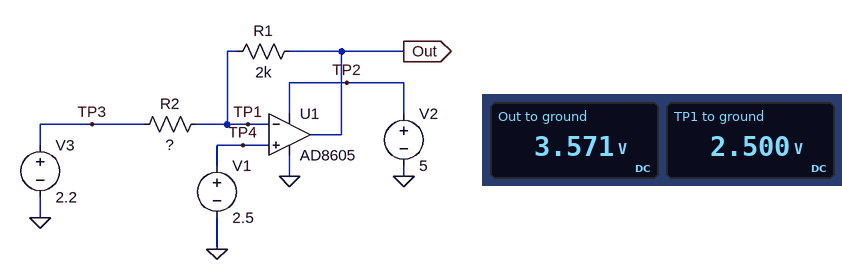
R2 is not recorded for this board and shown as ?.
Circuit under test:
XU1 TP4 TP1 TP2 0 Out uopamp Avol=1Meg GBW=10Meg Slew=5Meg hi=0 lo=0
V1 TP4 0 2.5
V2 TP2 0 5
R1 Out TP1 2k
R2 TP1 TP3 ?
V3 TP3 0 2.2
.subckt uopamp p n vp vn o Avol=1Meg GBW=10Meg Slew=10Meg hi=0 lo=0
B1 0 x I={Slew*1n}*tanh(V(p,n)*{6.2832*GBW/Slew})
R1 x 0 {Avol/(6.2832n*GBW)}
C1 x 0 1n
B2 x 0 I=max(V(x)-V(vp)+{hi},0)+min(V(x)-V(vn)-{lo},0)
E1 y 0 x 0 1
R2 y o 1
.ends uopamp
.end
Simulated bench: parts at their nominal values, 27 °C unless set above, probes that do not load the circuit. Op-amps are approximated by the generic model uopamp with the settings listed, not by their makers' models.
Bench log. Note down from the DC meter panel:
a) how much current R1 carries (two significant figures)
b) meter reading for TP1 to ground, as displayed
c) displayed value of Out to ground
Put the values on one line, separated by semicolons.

540 µA; 2.500 V; 3.571 V
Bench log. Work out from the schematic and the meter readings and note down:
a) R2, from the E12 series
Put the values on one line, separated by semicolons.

560 Ω
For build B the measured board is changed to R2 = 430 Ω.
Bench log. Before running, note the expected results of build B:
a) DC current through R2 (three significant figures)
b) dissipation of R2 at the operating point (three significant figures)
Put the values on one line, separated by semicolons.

698 µA; 209 µW
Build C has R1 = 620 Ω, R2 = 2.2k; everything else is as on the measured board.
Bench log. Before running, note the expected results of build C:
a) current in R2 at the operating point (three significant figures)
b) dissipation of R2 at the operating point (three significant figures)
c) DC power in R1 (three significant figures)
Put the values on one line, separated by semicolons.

136 µA; 40.9 µW; 11.5 µW
